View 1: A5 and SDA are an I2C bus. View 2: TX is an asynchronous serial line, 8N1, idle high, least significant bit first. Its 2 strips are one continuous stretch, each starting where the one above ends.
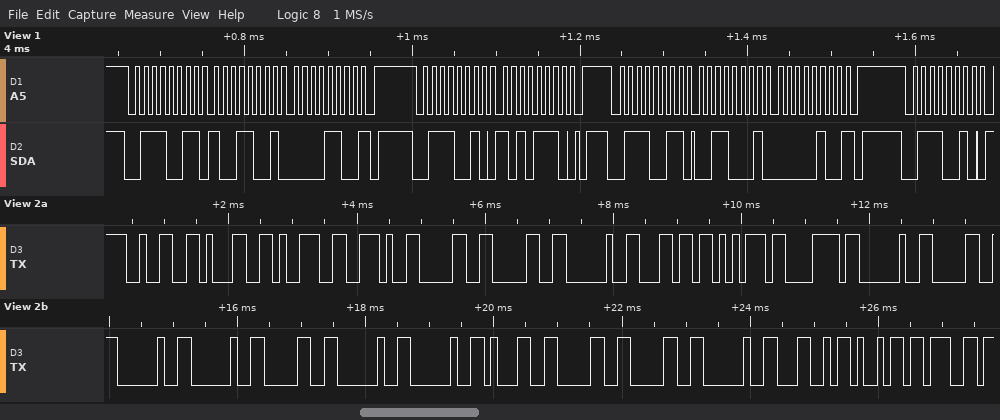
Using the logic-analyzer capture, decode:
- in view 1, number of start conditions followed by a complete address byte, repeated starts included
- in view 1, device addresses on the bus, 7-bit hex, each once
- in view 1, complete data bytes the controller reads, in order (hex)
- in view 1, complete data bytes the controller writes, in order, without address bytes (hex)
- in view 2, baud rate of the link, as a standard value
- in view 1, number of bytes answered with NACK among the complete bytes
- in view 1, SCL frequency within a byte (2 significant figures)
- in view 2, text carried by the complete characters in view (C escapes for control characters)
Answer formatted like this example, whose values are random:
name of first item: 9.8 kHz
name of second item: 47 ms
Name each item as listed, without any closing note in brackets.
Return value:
in view 1, number of start conditions followed by a complete address byte, repeated starts included: 4
in view 1, device addresses on the bus, 7-bit hex, each once: 0x39
in view 1, complete data bytes the controller reads, in order: 99 0C 31 04
in view 1, complete data bytes the controller writes, in order, without address bytes: AE
in view 2, baud rate of the link, as a standard value: 9600 baud
in view 1, number of bytes answered with NACK among the complete bytes: 2
in view 1, SCL frequency within a byte: 100 kHz
in view 2, text carried by the complete characters in view: "219.00 lux 0  0  100 Lig"
